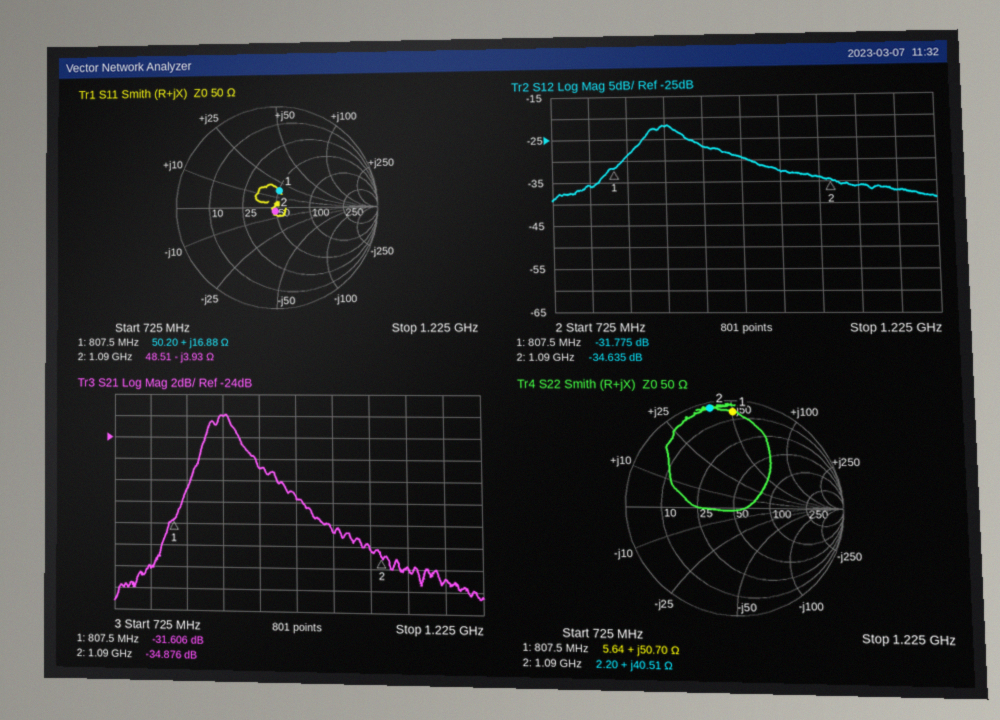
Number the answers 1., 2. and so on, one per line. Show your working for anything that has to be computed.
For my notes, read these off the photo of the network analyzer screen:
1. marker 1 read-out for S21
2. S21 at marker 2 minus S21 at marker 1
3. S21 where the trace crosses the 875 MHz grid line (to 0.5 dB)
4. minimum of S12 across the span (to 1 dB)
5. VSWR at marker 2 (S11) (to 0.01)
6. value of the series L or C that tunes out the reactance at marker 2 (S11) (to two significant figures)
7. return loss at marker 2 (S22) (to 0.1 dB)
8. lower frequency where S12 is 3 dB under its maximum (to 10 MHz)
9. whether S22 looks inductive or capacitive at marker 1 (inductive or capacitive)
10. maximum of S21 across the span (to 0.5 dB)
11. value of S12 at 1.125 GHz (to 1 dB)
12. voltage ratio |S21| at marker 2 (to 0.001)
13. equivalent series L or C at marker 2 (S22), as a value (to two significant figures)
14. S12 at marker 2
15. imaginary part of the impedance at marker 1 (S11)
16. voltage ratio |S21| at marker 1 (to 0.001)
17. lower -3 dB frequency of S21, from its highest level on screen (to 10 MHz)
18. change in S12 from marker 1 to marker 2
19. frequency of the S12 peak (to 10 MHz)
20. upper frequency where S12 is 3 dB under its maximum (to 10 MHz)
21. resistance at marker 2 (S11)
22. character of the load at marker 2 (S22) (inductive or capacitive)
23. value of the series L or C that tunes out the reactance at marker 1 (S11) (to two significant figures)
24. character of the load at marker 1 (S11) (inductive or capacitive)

1. -31.606 dB
2. -34.876 − (-31.606) = -3.270 dB
3. -22.0 dB
4. -39 dB
5. 1.09
6. L = 3.93 Ω/(2π × 1.09 GHz) ≈ 574 pH, so 570 pH to two significant figures
7. 0.5 dB
8. 850 MHz
9. inductive
10. -22.0 dB
11. -36 dB
12. 10^(-34.876/20) ≈ 0.018
13. L = 40.51 Ω/(2π × 1.09 GHz) ≈ 5.9 nH
14. -34.635 dB
15. +16.88 Ω
16. 10^(-31.606/20) ≈ 0.026
17. 850 MHz
18. -34.635 − (-31.775) = -2.860 dB
19. 880 MHz
20. 900 MHz
21. 48.51 Ω
22. inductive
23. C = 1/(2π × 807.5 MHz × 16.88 Ω) ≈ 12 pF
24. inductive
